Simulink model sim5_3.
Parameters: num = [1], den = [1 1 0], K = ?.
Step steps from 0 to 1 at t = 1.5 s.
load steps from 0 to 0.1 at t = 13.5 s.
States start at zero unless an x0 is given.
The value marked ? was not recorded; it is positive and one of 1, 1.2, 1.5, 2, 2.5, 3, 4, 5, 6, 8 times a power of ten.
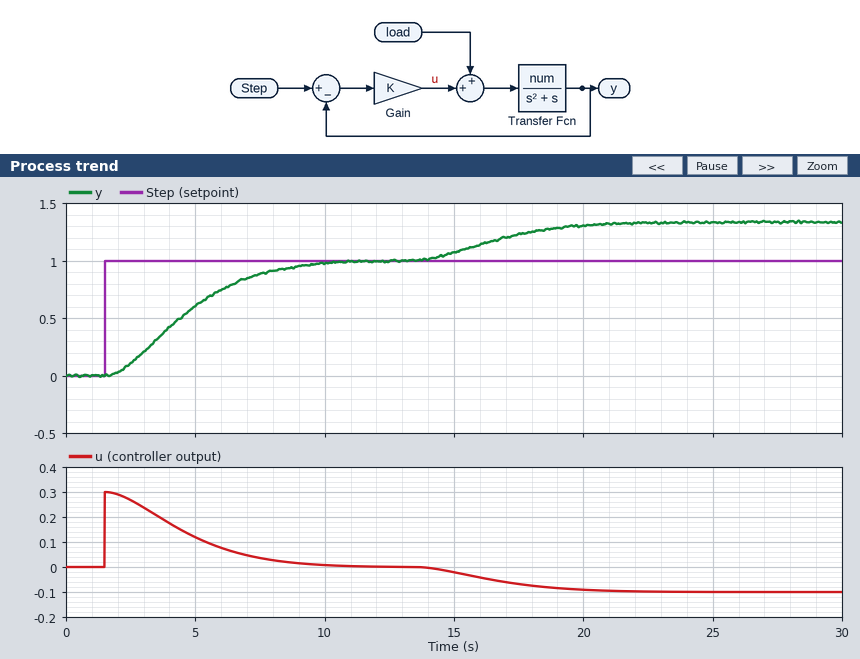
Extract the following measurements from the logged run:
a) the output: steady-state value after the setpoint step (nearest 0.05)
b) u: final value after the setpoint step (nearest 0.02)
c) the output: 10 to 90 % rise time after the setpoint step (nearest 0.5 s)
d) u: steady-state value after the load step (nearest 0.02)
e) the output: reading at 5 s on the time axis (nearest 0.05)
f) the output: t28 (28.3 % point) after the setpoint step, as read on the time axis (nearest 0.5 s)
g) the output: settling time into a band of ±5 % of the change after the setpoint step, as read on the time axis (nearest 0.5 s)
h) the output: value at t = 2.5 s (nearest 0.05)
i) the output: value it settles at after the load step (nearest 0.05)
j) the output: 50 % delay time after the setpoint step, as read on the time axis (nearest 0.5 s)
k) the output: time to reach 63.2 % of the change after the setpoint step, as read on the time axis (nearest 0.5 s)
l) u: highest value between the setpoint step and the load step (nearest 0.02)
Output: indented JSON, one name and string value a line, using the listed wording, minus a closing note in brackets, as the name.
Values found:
{
  "the output: steady-state value after the setpoint step": "1.00",
  "u: final value after the setpoint step": "0.00",
  "the output: 10 to 90 % rise time after the setpoint step": "5.5 s",
  "u: steady-state value after the load step": "-0.10",
  "the output: reading at 5 s on the time axis": "0.60",
  "the output: t28 (28.3 % point) after the setpoint step, as read on the time axis": "3.5 s",
  "the output: settling time into a band of ±5 % of the change after the setpoint step, as read on the time axis": "9.0 s",
  "the output: value at t = 2.5 s": "0.10",
  "the output: value it settles at after the load step": "1.35",
  "the output: 50 % delay time after the setpoint step, as read on the time axis": "4.5 s",
  "the output: time to reach 63.2 % of the change after the setpoint step, as read on the time axis": "5.0 s",
  "u: highest value between the setpoint step and the load step": "0.30"
}
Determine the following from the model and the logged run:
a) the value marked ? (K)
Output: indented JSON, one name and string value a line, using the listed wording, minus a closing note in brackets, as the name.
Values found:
{
  "the value marked ?": "0.3"
}
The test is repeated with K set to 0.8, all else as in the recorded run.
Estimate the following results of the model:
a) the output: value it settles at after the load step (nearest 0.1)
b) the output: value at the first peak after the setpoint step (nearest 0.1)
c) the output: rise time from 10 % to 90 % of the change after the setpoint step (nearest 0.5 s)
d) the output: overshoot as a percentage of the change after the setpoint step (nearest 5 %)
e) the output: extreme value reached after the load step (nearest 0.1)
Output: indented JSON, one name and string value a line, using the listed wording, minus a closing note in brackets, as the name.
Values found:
{
  "the output: value it settles at after the load step": "1.1",
  "the output: value at the first peak after the setpoint step": "1.1",
  "the output: rise time from 10 % to 90 % of the change after the setpoint step": "2.0 s",
  "the output: overshoot as a percentage of the change after the setpoint step": "10 %",
  "the output: extreme value reached after the load step": "1.1"
}
